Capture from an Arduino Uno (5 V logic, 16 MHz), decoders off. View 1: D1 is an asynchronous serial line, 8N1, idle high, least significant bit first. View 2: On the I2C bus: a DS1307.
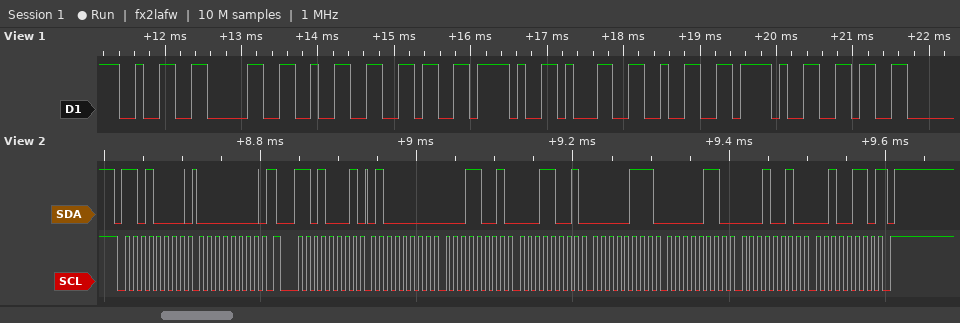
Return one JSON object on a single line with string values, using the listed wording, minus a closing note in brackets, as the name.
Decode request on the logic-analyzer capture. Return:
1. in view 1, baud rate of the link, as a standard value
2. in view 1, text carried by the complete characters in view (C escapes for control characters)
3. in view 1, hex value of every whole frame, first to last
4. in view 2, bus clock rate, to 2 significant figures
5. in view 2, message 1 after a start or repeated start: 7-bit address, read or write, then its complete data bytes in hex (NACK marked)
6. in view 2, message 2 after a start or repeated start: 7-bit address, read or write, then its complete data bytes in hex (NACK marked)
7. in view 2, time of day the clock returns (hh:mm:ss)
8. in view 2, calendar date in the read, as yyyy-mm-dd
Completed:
{"in view 1, baud rate of the link, as a standard value": "9600 baud", "in view 1, text carried by the complete characters in view": "\"2026/12/6\"", "in view 1, hex value of every whole frame, first to last": "0x32 0x30 0x32 0x36 0x2F 0x31 0x32 0x2F 0x36", "in view 2, bus clock rate, to 2 significant figures": "100 kHz", "in view 2, message 1 after a start or repeated start: 7-bit address, read or write, then its complete data bytes in hex": "0x68 write: 00", "in view 2, message 2 after a start or repeated start: 7-bit address, read or write, then its complete data bytes in hex": "0x68 read: 40 19 19 07 06 12 26 NACK", "in view 2, time of day the clock returns": "19:19:40", "in view 2, calendar date in the read, as yyyy-mm-dd": "2026-12-06"}
